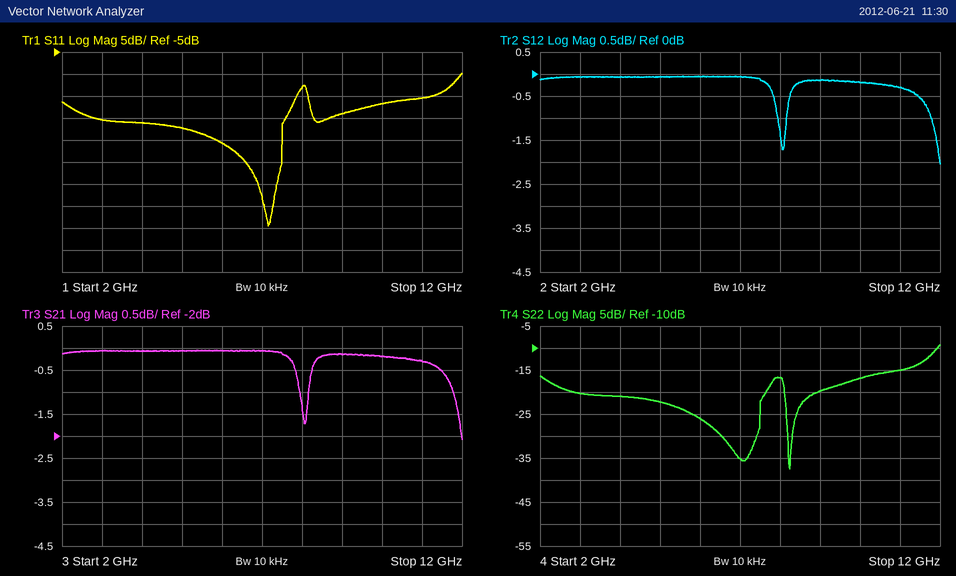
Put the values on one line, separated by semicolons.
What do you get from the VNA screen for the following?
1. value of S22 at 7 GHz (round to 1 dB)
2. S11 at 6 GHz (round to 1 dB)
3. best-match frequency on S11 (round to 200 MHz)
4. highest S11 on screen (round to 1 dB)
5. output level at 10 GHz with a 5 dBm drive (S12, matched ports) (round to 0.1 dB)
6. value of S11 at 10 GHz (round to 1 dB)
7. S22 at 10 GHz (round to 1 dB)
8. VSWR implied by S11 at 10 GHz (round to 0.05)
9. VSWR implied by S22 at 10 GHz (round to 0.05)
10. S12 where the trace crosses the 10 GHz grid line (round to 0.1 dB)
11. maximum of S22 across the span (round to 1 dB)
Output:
-35 dB; -26 dB; 7.2 GHz; -10 dB; 4.8 dBm; -17 dB; -17 dB; 1.35; 1.35; -0.2 dB; -9 dB
